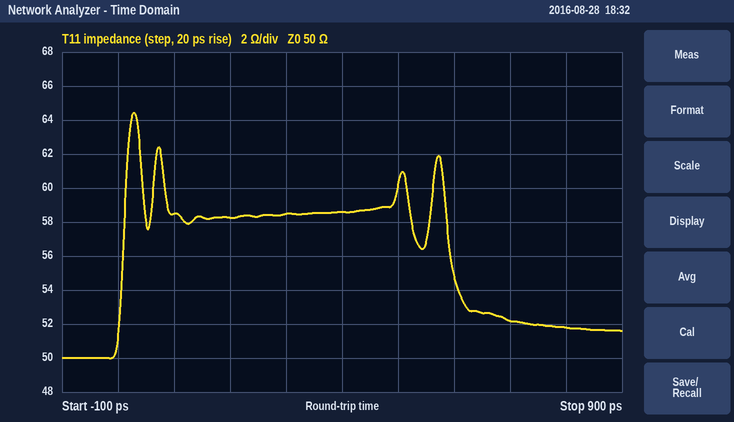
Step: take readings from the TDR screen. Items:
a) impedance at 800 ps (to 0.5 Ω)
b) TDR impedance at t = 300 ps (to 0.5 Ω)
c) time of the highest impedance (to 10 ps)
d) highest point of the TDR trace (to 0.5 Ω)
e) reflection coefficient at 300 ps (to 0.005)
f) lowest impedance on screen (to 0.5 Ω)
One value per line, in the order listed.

52.0 Ω
58.5 Ω
30 ps
64.5 Ω
+0.080
50.0 Ω
